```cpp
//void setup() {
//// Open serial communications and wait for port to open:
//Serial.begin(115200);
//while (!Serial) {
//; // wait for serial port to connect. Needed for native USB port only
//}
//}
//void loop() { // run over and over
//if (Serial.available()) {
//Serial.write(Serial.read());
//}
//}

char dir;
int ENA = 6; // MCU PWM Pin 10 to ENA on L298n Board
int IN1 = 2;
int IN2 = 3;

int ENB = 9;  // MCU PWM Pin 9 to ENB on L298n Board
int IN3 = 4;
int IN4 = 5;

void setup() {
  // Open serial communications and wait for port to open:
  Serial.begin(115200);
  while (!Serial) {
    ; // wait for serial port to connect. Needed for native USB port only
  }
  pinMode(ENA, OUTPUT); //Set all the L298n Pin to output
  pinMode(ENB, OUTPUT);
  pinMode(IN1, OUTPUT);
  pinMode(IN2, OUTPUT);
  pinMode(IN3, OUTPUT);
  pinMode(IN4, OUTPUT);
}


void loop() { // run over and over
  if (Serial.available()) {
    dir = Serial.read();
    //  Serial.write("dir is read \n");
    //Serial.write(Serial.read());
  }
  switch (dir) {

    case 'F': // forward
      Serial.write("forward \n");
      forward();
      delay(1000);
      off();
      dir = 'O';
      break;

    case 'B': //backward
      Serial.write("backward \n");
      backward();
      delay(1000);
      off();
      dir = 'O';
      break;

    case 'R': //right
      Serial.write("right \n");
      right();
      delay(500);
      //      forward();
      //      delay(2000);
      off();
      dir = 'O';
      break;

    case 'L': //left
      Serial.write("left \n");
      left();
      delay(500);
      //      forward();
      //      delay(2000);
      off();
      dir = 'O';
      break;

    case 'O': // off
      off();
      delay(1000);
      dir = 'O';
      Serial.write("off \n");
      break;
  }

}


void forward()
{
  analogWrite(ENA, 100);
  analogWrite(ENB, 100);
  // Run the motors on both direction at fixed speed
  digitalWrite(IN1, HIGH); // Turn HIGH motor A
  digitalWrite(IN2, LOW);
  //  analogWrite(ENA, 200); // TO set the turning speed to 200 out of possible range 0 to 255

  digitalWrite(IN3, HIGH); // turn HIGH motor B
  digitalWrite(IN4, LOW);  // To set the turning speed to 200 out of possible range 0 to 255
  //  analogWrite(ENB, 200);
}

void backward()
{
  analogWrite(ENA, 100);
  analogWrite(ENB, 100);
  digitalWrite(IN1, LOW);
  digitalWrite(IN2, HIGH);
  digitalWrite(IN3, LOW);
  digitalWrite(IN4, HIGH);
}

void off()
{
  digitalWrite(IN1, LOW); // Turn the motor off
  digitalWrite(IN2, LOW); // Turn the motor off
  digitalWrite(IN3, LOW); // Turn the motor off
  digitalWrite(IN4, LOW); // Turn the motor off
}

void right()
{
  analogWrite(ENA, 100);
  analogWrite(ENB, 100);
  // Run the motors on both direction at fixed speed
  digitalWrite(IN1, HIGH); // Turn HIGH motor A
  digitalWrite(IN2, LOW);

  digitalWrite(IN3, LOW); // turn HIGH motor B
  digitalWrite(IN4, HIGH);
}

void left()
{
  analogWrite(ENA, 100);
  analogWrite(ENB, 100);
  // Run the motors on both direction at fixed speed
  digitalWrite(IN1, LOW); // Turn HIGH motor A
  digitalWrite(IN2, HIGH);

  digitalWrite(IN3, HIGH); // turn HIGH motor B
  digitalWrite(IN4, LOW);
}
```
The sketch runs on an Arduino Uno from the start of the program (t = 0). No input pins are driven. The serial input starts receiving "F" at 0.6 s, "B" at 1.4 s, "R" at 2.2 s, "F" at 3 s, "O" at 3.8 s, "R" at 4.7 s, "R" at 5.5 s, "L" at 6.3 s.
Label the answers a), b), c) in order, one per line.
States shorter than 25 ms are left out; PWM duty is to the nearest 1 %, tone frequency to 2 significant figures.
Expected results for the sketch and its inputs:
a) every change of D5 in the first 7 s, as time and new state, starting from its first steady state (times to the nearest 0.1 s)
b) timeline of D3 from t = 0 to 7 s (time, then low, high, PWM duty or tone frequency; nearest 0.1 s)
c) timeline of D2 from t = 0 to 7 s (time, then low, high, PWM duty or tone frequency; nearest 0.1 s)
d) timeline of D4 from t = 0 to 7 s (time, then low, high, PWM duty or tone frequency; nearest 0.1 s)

a) 0 s low; 1.6 s high; 3.1 s low; 5.1 s high; 6.1 s low
b) 0 s low; 1.6 s high; 2.6 s low
c) 0 s low; 0.6 s high; 1.6 s low; 2.6 s high; 4.1 s low; 5.1 s high; 6.1 s low
d) 0 s low; 0.6 s high; 1.6 s low; 3.1 s high; 4.1 s low
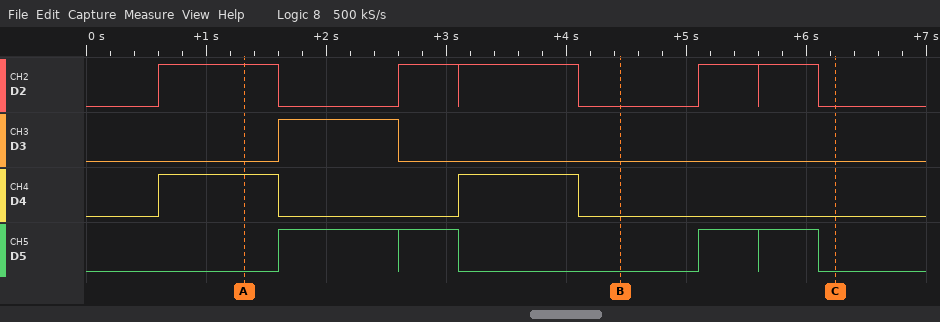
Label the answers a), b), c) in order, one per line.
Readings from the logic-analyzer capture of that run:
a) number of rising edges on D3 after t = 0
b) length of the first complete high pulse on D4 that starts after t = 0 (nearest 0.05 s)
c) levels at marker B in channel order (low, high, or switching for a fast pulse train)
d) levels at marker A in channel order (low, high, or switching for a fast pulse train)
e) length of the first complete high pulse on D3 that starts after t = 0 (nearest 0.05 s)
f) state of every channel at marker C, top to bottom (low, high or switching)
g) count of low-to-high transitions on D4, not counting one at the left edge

a) 1
b) 1.00 s
c) D2 low, D3 low, D4 low, D5 low
d) D2 high, D3 low, D4 high, D5 low
e) 1.00 s
f) D2 low, D3 low, D4 low, D5 low
g) 2
